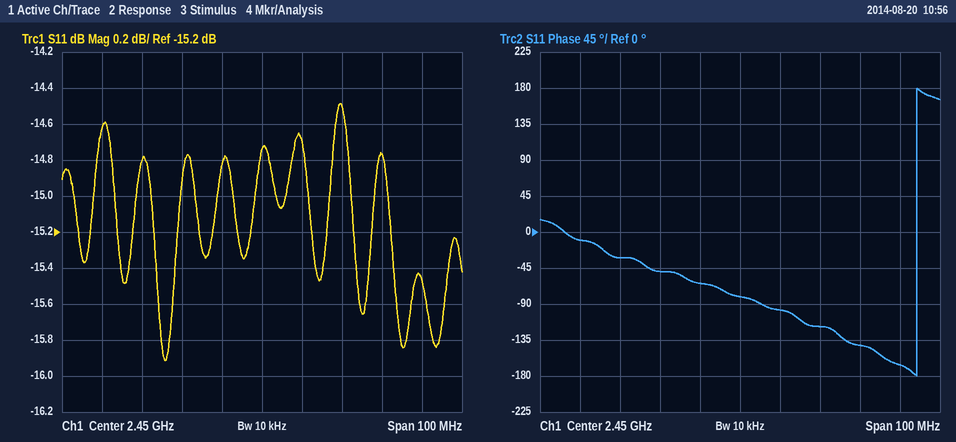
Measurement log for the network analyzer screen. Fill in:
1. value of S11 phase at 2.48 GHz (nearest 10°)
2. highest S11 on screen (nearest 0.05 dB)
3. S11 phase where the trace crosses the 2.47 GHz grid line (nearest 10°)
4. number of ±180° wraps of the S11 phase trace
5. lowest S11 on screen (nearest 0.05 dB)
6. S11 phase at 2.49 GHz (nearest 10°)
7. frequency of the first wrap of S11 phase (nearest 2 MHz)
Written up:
-140°
-14.50 dB
-120°
1
-15.90 dB
-170°
2.494 GHz
